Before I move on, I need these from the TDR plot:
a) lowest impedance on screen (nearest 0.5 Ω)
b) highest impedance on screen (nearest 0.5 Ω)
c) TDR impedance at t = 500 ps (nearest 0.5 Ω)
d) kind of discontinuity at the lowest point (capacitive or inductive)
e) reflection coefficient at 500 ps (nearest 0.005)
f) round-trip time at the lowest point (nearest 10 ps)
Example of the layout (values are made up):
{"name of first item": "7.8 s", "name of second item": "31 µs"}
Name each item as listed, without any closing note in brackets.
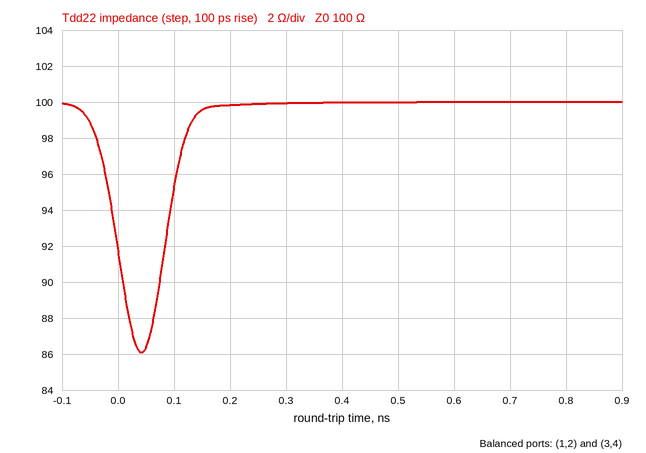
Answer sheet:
{"lowest impedance on screen": "86.0 Ω", "highest impedance on screen": "100.0 Ω", "TDR impedance at t = 500 ps": "100.0 Ω", "kind of discontinuity at the lowest point": "capacitive", "reflection coefficient at 500 ps": "0.000", "round-trip time at the lowest point": "40 ps"}
